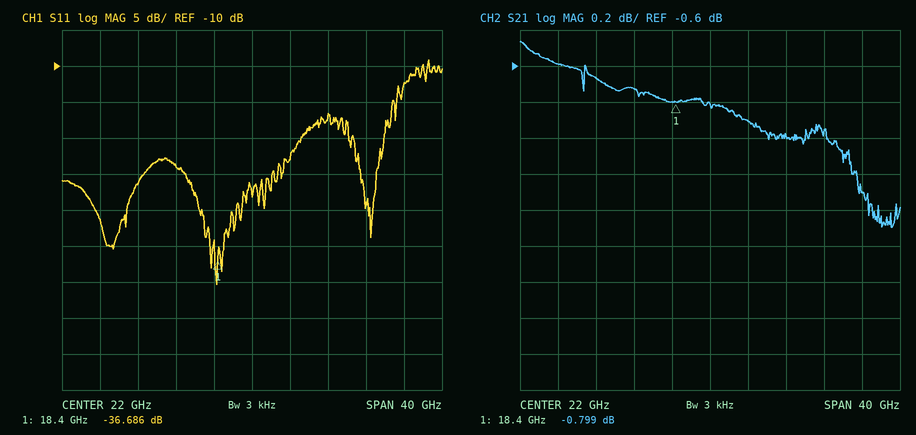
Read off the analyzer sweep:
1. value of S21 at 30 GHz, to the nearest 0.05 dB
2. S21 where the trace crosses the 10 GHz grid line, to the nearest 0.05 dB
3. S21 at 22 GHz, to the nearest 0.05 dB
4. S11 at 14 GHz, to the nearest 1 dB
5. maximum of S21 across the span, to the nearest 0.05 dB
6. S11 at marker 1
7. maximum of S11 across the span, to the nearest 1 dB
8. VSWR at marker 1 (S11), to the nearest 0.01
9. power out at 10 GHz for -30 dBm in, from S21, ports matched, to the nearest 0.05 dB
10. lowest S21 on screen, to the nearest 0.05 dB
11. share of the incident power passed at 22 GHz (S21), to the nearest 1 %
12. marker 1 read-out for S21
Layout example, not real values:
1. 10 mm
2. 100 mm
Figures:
1. -1.00 dB
2. -0.65 dB
3. -0.80 dB
4. -24 dB
5. -0.45 dB
6. -36.686 dB
7. -9 dB
8. 1.03
9. -30.65 dBm
10. -1.50 dB
11. 83 %
12. -0.799 dB
